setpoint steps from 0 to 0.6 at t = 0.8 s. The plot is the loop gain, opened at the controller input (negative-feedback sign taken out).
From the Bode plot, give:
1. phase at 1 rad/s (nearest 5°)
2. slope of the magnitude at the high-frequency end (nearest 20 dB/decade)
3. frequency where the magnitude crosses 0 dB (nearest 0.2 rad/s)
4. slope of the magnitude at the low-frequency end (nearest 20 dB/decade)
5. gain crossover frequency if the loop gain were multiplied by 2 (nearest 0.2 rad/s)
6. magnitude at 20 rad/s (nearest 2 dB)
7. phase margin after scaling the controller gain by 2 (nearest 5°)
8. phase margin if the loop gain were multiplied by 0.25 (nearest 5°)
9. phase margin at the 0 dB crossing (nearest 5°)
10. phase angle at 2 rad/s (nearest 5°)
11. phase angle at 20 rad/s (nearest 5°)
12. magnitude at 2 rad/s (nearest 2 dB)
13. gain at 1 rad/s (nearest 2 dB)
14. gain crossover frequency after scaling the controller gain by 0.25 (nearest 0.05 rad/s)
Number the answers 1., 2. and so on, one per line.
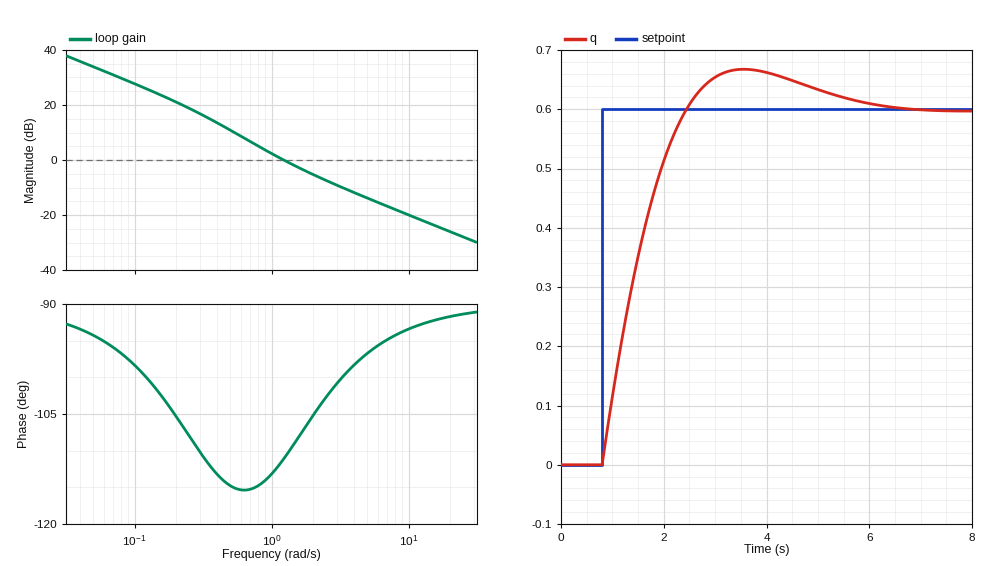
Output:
1. -115°
2. -20 dB/decade
3. 1.2 rad/s
4. -20 dB/decade
5. 2.2 rad/s
6. -26 dB
7. 75°
8. 65°
9. 70°
10. -105°
11. -90°
12. -6 dB
13. 2 dB
14. 0.45 rad/s
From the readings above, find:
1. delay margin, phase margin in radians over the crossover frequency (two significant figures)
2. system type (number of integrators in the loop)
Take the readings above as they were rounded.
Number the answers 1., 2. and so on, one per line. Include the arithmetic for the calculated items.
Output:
1. 70 × π / 180 / 1.2 = 1.0 s
2. 1
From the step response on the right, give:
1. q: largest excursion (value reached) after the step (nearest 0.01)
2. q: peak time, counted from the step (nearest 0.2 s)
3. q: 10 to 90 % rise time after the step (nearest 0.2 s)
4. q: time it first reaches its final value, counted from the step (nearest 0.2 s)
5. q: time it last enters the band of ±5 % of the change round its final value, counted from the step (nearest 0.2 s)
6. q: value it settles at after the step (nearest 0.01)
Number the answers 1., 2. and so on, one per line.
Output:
1. 0.67
2. 2.8 s
3. 1.2 s
4. 1.6 s
5. 4.4 s
6. 0.60
